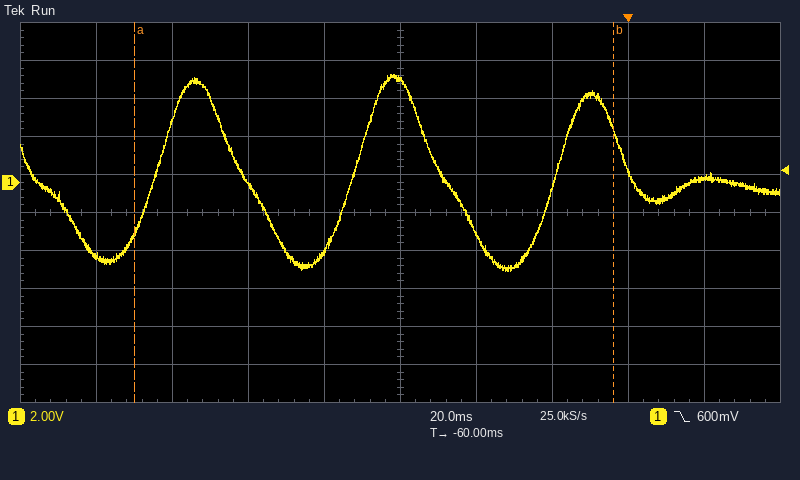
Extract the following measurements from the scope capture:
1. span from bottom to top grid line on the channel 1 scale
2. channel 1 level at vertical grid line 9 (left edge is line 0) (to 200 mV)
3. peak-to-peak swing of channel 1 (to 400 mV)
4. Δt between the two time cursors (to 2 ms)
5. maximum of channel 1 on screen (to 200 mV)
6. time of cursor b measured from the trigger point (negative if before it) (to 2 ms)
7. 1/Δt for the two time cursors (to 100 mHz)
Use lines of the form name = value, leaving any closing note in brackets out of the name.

span from bottom to top grid line on the channel 1 scale = 20 V
channel 1 level at vertical grid line 9 (left edge is line 0) = 200 mV
peak-to-peak swing of channel 1 = 10.4 V
Δt between the two time cursors = 126 ms
maximum of channel 1 on screen = 5.6 V
time of cursor b measured from the trigger point (negative if before it) = -4 ms
1/Δt for the two time cursors = 7.9 Hz
